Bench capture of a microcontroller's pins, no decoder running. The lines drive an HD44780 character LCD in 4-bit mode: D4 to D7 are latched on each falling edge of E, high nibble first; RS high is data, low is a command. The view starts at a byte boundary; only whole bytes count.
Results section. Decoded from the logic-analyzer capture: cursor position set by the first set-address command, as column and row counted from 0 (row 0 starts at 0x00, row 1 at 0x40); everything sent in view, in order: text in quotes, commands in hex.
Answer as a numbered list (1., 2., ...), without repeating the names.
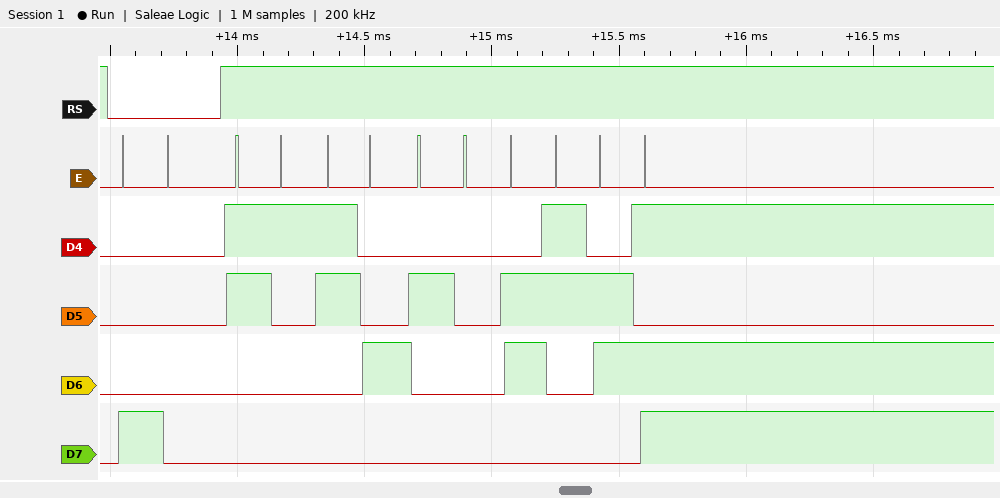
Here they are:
1. column 0, row 0
2. 0x80 "14 cm"
